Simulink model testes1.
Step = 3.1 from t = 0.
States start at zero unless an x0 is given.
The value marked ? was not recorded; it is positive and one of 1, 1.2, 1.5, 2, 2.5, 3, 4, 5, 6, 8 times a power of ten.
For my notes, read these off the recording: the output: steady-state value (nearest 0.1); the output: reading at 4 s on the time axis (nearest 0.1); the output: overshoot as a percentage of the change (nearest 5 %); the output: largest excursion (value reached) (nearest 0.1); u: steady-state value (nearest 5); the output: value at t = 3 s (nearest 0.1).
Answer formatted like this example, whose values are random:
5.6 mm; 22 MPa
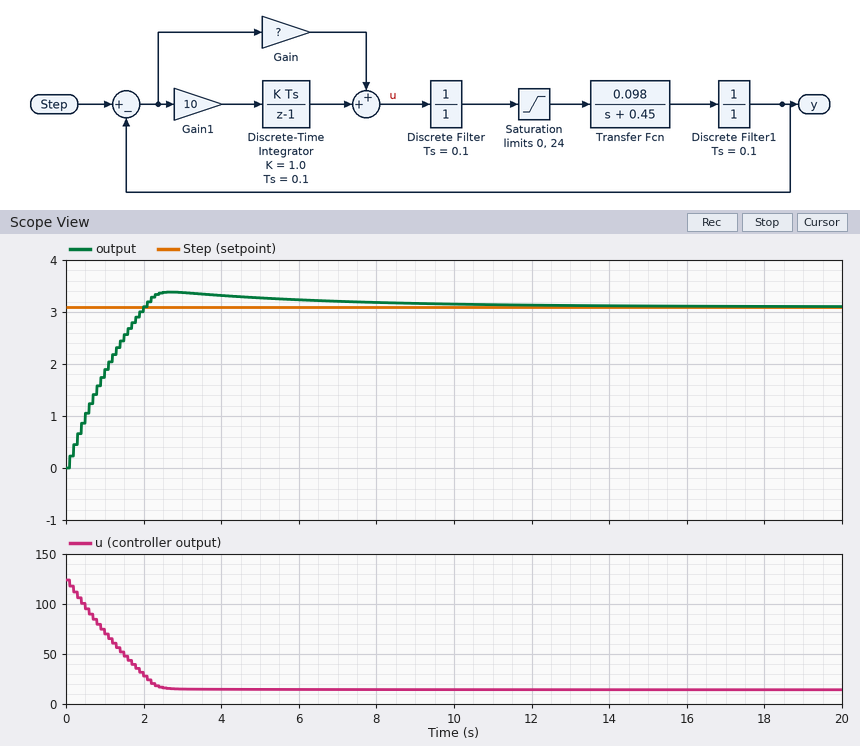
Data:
3.1; 3.3; 10 %; 3.4; 15; 3.4
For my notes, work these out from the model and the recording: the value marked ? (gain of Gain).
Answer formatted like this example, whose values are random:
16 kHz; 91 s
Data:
40
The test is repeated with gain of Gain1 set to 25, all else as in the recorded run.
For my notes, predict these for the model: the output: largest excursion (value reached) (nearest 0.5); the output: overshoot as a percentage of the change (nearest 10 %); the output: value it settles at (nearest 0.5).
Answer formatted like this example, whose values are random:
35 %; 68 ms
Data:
4.0; 30 %; 3.0
